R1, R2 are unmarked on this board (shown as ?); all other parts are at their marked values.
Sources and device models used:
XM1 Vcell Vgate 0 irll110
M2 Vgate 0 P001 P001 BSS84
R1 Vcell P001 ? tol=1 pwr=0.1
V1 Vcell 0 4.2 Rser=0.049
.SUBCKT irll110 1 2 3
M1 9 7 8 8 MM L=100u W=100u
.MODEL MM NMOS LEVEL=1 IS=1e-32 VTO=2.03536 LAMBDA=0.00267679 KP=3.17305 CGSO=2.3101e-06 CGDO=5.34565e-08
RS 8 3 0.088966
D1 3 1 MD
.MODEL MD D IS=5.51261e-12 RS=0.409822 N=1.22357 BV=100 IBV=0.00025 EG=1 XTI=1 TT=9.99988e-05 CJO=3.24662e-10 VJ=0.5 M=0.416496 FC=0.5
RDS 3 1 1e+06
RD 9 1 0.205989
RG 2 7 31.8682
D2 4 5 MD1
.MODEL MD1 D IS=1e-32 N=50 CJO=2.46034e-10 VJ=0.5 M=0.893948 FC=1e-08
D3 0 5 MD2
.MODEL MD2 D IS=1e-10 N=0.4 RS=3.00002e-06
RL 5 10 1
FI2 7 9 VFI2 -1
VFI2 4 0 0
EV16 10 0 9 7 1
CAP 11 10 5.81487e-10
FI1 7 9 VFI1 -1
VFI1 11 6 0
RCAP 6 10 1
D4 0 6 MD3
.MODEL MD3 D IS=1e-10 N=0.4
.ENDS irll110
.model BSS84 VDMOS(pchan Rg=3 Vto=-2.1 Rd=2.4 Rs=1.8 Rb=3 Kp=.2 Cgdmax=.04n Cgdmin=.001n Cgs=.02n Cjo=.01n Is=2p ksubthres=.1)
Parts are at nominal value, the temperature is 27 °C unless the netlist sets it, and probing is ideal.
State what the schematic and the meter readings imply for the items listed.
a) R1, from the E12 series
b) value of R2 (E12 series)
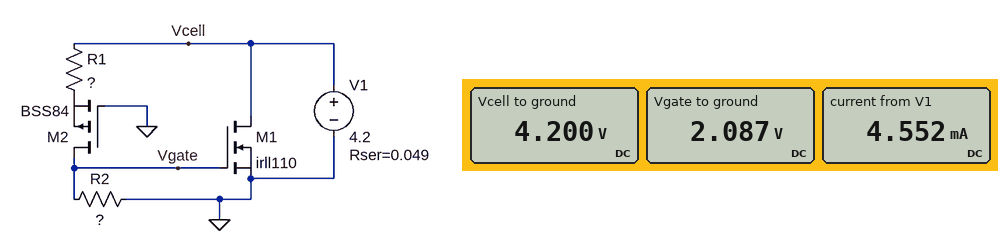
6.8 kΩ
6.8 kΩ
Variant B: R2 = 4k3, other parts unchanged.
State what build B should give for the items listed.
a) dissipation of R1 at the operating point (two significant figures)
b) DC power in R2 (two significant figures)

670 µW
420 µW
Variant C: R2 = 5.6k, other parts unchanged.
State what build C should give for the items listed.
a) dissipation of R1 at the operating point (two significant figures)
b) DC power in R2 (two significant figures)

670 µW
550 µW
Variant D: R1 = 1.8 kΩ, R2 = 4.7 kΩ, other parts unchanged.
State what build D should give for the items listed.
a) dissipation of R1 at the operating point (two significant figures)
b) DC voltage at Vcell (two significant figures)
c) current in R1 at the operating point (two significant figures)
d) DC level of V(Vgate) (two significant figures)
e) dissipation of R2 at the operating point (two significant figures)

730 µW
4.1 V
640 µA
3.0 V
1.9 mW
